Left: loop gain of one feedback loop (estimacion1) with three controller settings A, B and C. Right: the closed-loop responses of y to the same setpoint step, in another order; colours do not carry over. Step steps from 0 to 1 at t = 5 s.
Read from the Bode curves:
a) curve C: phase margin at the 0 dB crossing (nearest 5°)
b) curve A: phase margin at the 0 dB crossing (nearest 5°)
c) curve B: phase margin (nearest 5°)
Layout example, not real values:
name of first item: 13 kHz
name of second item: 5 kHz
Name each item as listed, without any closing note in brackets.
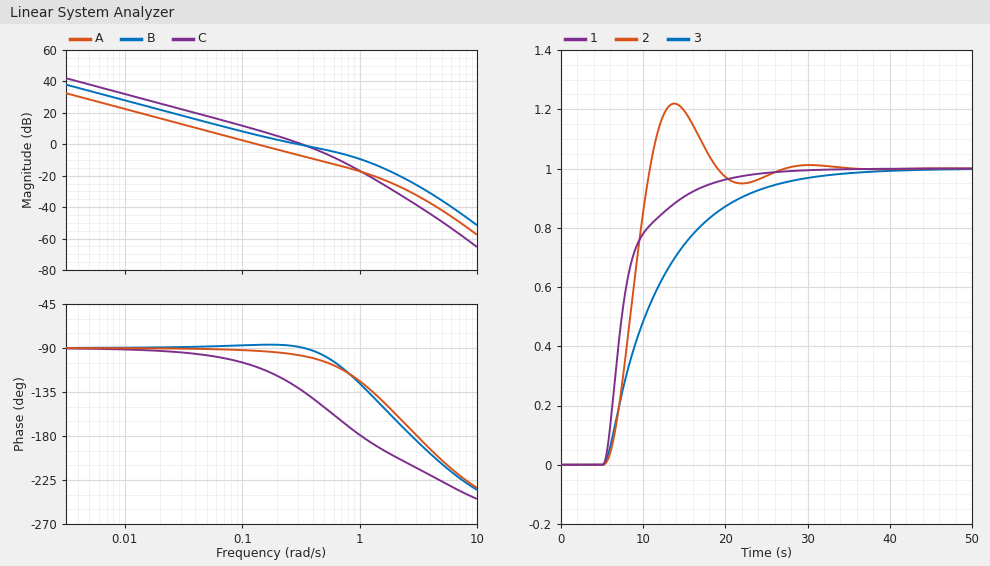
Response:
curve C: phase margin at the 0 dB crossing: 45°
curve A: phase margin at the 0 dB crossing: 85°
curve B: phase margin: 90°
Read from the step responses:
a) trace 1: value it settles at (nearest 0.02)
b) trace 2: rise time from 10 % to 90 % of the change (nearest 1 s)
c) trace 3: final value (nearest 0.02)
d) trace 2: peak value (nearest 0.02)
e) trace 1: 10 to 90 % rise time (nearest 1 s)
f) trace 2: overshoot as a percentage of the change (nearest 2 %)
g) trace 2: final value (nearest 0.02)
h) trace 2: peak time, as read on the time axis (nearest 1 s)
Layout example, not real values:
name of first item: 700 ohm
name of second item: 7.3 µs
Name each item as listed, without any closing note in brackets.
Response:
trace 1: value it settles at: 1.00
trace 2: rise time from 10 % to 90 % of the change: 4 s
trace 3: final value: 1.00
trace 2: peak value: 1.22
trace 1: 10 to 90 % rise time: 9 s
trace 2: overshoot as a percentage of the change: 22 %
trace 2: final value: 1.00
trace 2: peak time, as read on the time axis: 14 s
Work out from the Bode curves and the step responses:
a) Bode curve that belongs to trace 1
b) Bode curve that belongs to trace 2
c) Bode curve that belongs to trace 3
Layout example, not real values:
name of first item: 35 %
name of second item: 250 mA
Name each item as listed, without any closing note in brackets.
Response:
Bode curve that belongs to trace 1: B
Bode curve that belongs to trace 2: C
Bode curve that belongs to trace 3: A
